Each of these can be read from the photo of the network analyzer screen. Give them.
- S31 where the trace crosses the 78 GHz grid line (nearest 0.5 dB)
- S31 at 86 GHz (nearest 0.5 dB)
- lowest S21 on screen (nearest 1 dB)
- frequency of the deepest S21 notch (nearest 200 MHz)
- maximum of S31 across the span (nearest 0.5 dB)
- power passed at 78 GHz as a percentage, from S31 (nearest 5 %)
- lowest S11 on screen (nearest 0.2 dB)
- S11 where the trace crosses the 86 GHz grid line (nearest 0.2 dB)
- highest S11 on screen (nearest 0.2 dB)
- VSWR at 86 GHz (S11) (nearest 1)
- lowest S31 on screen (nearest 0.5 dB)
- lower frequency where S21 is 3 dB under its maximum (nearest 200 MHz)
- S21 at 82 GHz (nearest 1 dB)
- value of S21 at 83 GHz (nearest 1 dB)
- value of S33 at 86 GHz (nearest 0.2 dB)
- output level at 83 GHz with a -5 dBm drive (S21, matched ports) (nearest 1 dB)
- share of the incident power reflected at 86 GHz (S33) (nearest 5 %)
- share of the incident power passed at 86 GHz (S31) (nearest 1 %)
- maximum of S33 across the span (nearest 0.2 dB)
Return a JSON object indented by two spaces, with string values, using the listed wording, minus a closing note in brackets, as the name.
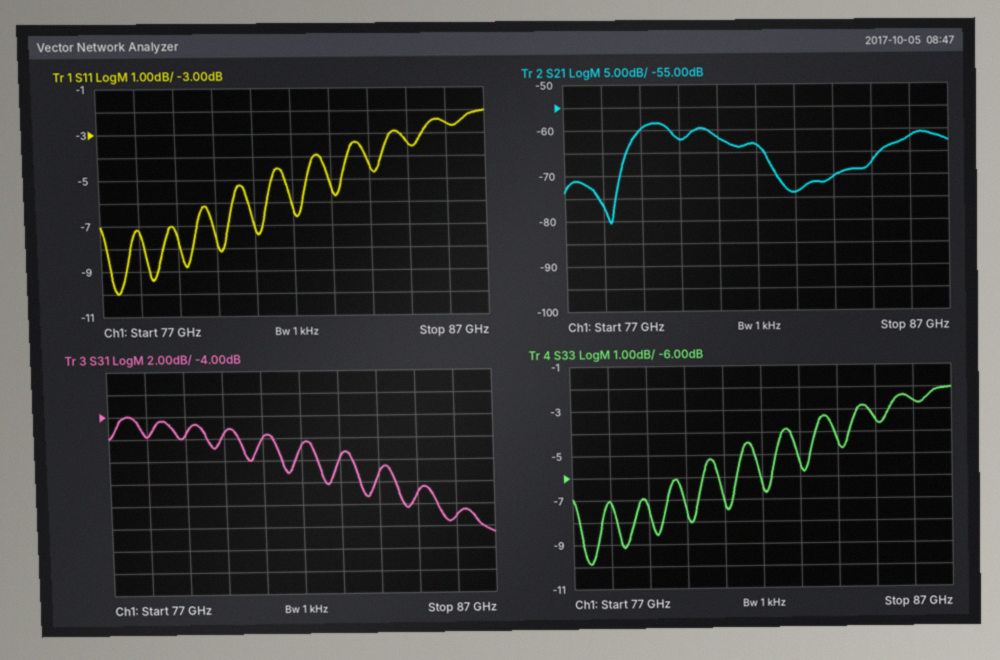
{
  "S31 where the trace crosses the 78 GHz grid line": "-6.0 dB",
  "S31 at 86 GHz": "-13.0 dB",
  "lowest S21 on screen": "-80 dB",
  "frequency of the deepest S21 notch": "78.2 GHz",
  "maximum of S31 across the span": "-4.0 dB",
  "power passed at 78 GHz as a percentage, from S31": "25 %",
  "lowest S11 on screen": "-10.0 dB",
  "S11 where the trace crosses the 86 GHz grid line": "-2.6 dB",
  "highest S11 on screen": "-2.0 dB",
  "VSWR at 86 GHz (S11)": "7",
  "lowest S31 on screen": "-14.5 dB",
  "lower frequency where S21 is 3 dB under its maximum": "78.8 GHz",
  "S21 at 82 GHz": "-63 dB",
  "value of S21 at 83 GHz": "-74 dB",
  "value of S33 at 86 GHz": "-2.6 dB",
  "output level at 83 GHz with a -5 dBm drive (S21, matched ports)": "-79 dBm",
  "share of the incident power reflected at 86 GHz (S33)": "55 %",
  "share of the incident power passed at 86 GHz (S31)": "5 %",
  "maximum of S33 across the span": "-2.0 dB"
}
